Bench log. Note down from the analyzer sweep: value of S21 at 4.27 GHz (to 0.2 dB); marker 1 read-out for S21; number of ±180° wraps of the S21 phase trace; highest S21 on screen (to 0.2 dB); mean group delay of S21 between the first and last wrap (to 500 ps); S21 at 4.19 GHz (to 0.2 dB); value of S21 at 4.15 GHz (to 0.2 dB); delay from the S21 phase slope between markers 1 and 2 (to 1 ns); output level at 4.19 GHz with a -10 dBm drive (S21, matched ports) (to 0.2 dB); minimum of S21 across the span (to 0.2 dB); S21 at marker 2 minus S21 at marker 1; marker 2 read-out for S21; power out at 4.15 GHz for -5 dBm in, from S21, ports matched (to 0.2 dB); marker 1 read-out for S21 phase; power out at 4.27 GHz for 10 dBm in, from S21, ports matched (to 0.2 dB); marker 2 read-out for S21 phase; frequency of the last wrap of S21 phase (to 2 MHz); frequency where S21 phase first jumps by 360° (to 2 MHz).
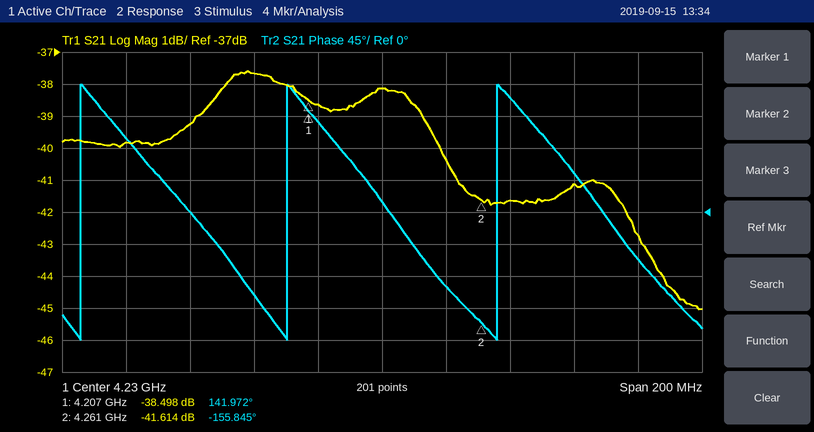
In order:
-41.6 dB
-38.498 dB
3
-37.6 dB
15.5 ns
-37.6 dB
-39.8 dB
15 ns
-47.6 dBm
-45.0 dB
-3.116 dB
-41.614 dB
-44.8 dBm
141.972°
-31.6 dBm
-155.845°
4.266 GHz
4.136 GHz
